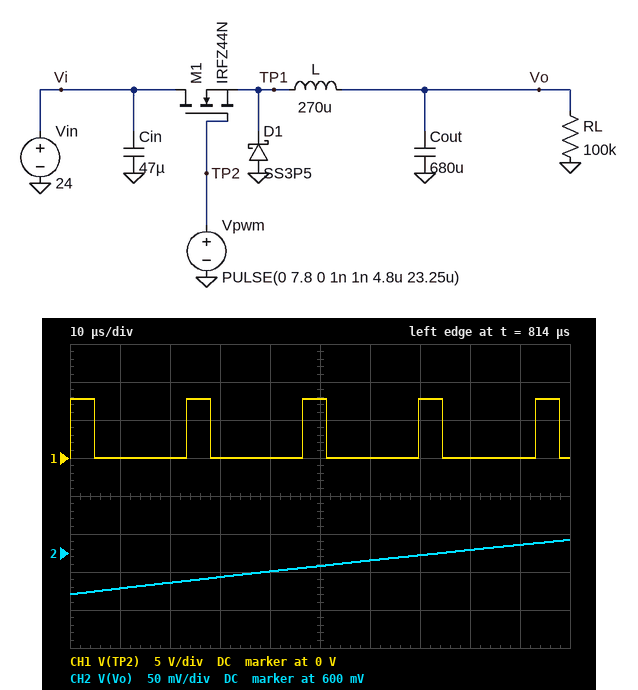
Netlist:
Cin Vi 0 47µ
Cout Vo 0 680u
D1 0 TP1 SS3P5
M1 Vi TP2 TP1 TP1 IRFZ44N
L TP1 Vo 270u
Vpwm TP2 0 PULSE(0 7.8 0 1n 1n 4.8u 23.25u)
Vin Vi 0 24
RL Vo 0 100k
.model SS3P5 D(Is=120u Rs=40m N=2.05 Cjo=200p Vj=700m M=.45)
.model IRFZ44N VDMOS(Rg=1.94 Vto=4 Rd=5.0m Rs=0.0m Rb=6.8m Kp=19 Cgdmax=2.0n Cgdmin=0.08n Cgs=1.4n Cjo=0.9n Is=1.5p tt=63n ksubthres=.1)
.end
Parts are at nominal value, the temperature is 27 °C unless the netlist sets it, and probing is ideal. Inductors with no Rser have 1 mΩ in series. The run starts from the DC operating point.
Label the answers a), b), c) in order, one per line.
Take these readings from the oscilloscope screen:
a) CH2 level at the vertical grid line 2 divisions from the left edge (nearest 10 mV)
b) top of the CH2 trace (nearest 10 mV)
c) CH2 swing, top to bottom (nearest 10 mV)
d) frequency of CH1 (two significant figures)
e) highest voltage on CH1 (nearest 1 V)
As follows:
a) 560 mV
b) 620 mV
c) 70 mV
d) 43 kHz
e) 8 V
